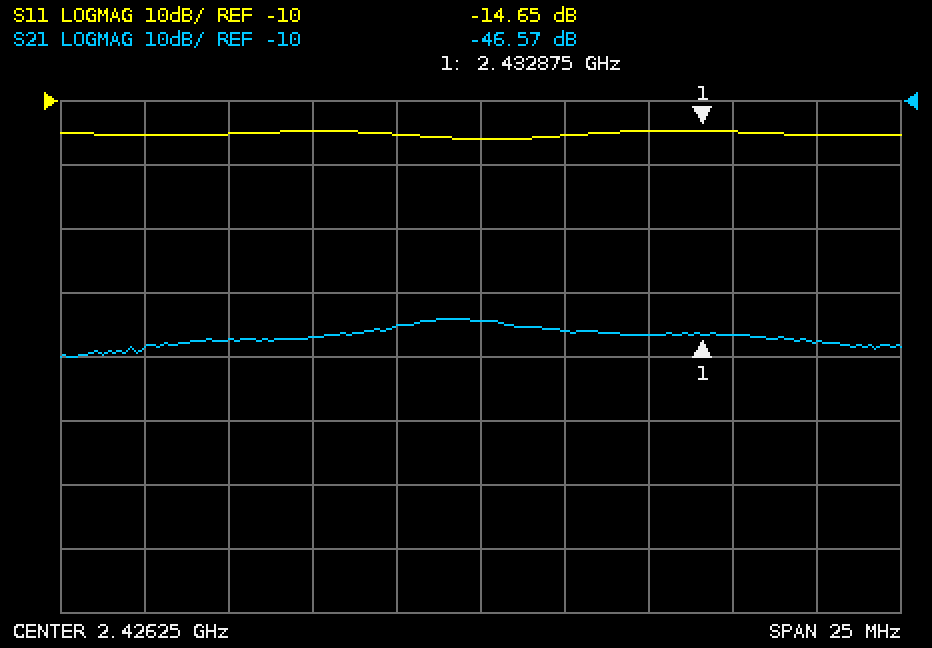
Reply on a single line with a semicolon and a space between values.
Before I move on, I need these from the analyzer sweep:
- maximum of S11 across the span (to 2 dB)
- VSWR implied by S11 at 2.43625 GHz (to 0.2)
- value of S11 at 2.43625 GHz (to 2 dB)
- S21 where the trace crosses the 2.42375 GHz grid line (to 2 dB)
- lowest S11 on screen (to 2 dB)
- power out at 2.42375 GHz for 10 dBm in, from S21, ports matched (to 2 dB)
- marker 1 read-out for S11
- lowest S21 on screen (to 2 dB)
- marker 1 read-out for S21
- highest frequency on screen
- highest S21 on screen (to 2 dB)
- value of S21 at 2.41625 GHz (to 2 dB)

-14 dB; 1.4; -16 dB; -46 dB; -16 dB; -36 dBm; -14.65 dB; -50 dB; -46.57 dB; 2.43875 GHz; -44 dB; -48 dB
